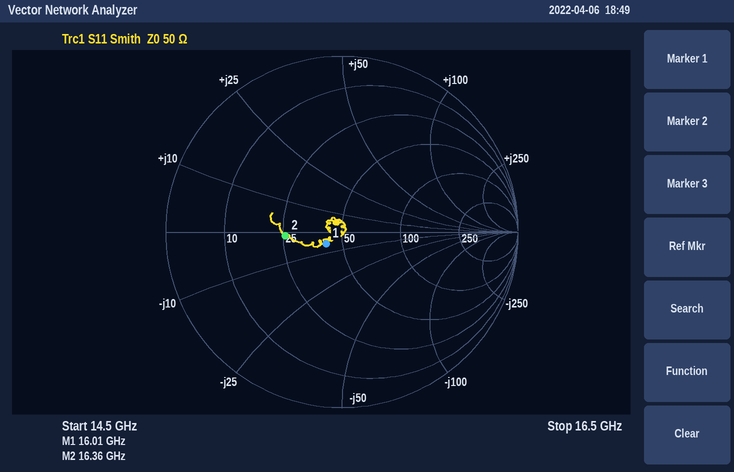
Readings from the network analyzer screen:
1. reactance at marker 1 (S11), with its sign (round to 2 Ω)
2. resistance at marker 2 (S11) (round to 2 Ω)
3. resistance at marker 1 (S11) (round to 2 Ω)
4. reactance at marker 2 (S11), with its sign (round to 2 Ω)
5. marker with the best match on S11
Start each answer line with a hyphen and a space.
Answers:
- -6 Ω
- 26 Ω
- 42 Ω
- -2 Ω
- marker 1
